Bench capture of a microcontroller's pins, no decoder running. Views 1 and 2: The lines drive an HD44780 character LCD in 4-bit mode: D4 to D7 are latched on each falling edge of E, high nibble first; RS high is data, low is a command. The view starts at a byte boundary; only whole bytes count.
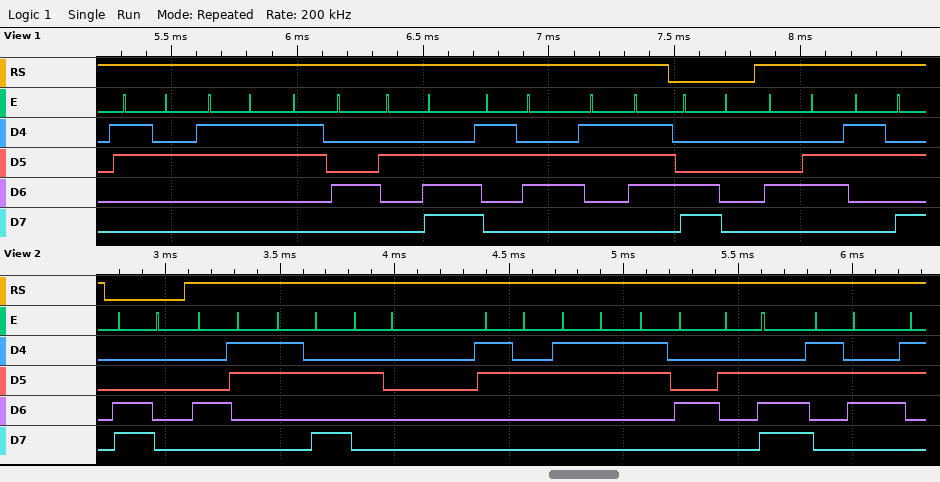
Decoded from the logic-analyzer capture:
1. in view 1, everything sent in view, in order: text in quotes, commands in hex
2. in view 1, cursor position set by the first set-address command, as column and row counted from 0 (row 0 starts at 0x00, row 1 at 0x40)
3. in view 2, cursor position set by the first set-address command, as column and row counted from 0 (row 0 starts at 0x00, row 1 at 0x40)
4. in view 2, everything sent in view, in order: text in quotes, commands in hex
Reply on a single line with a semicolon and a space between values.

"234.67" 0xC0 "F:"; column 0, row 1; column 0, row 1; 0xC0 "C: 234.6"
